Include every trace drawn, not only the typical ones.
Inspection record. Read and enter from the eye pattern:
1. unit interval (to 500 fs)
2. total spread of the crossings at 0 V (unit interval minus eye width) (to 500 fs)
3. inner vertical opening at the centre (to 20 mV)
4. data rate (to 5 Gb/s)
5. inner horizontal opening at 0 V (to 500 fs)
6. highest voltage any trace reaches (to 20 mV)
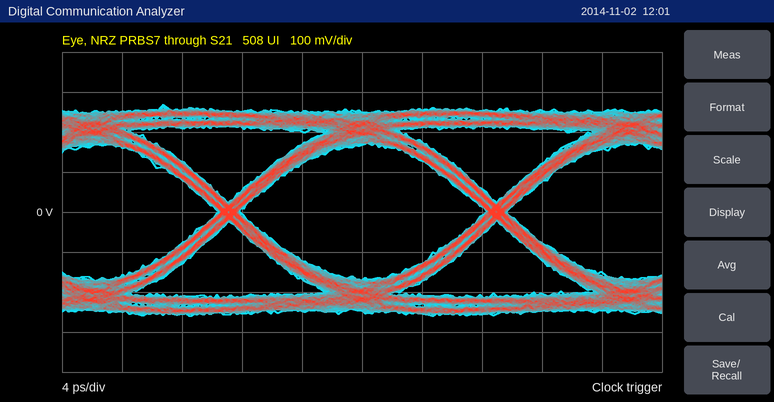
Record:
18.0 ps
1.5 ps
340 mV
55 Gb/s
16.5 ps
260 mV
